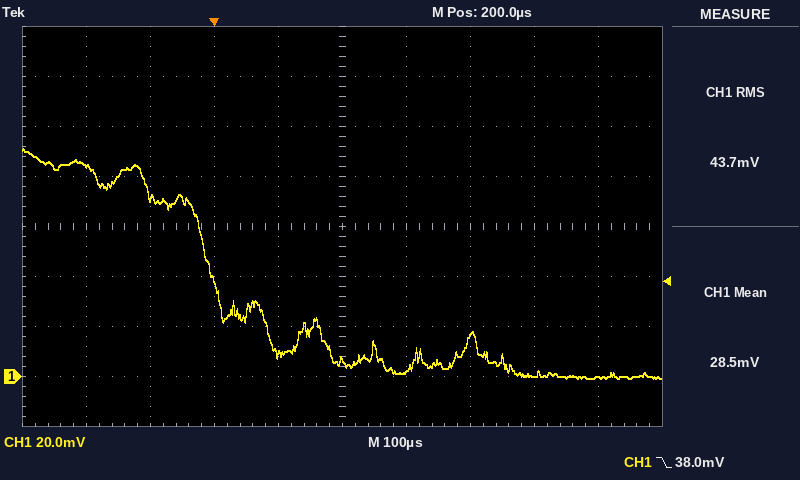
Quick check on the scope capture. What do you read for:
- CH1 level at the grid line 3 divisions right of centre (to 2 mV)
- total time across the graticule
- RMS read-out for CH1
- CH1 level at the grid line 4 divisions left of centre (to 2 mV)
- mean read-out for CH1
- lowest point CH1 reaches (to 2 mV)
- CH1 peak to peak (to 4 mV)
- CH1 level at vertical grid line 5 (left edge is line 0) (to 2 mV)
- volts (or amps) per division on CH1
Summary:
0 mV
1 ms
43.7 mV
84 mV
28.5 mV
0 mV
92 mV
6 mV
20 mV
